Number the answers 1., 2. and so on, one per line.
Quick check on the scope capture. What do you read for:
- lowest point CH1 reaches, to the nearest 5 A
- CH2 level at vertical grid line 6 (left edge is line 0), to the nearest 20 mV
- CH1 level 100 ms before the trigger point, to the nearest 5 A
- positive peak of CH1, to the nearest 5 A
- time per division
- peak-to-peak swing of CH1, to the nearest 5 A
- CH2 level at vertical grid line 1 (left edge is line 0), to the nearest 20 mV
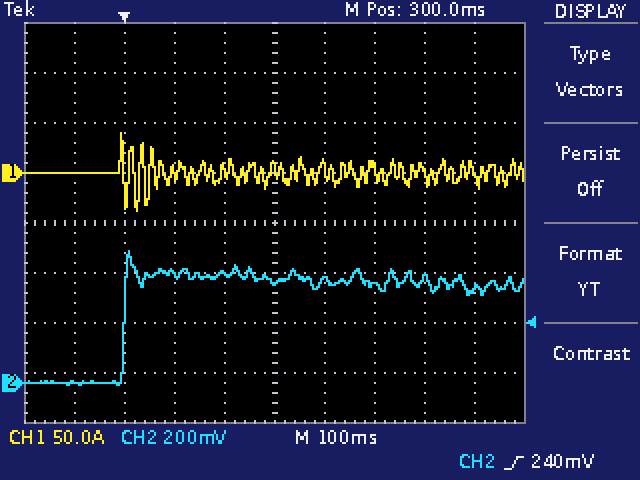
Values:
1. -40 A
2. 420 mV
3. 0 A
4. 40 A
5. 100 ms
6. 80 A
7. 0 mV
